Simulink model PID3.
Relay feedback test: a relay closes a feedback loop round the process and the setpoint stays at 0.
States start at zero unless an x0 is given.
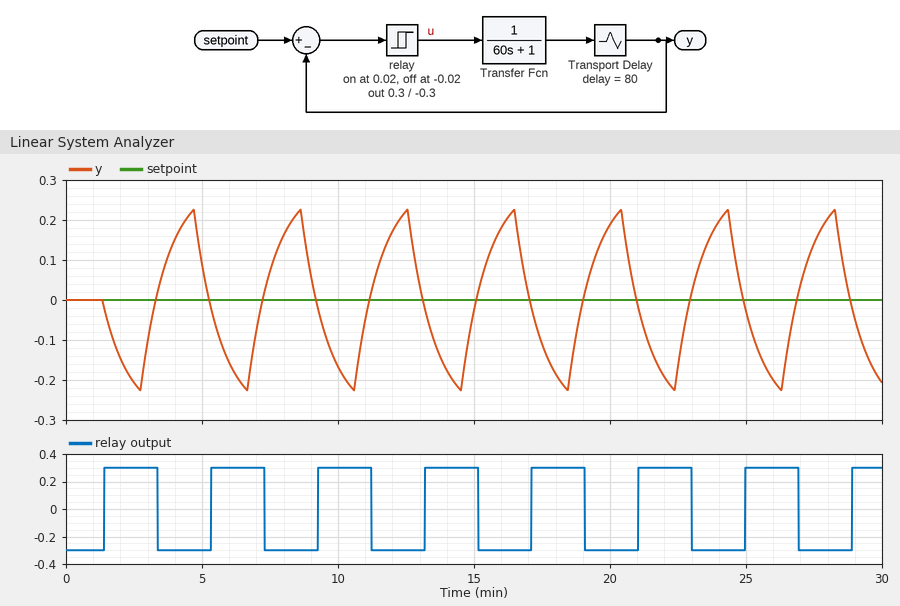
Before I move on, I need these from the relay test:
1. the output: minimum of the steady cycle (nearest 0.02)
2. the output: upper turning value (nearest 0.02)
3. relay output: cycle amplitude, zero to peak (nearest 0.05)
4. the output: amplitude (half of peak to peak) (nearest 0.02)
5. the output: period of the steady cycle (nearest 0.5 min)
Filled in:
-0.22
0.22
0.30
0.22
4.0 min
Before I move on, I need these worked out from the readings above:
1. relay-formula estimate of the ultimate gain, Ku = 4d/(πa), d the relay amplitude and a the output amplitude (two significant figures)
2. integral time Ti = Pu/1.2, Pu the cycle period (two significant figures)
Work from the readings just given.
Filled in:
1.7
3.3 min
